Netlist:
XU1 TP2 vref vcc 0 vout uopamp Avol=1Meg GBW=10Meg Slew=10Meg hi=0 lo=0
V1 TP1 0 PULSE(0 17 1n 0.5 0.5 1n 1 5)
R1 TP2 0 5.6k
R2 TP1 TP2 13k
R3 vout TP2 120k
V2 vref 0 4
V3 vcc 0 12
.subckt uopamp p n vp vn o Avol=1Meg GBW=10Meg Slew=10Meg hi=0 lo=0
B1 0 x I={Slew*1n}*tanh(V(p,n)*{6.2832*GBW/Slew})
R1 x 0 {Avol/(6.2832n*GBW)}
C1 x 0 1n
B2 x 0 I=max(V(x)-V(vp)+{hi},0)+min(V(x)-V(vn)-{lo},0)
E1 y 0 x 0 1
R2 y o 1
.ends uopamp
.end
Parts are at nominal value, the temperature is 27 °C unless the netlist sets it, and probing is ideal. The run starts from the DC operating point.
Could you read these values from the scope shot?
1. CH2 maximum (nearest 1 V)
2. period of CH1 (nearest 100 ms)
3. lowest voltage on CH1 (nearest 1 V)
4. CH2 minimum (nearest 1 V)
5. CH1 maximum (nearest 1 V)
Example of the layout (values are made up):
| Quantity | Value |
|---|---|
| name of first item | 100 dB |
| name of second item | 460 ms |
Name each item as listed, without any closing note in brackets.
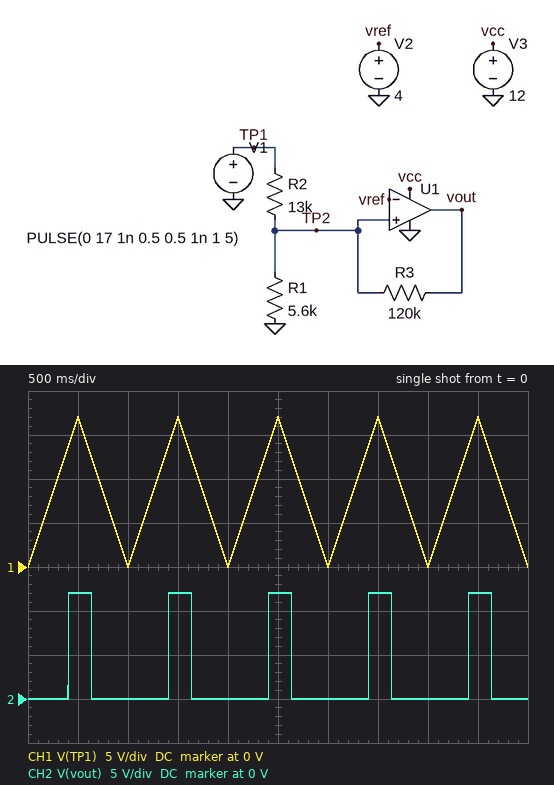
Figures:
| Quantity | Value |
|---|---|
| CH2 maximum | 12 V |
| period of CH1 | 1.0 s |
| lowest voltage on CH1 | 0 V |
| CH2 minimum | 0 V |
| CH1 maximum | 17 V |
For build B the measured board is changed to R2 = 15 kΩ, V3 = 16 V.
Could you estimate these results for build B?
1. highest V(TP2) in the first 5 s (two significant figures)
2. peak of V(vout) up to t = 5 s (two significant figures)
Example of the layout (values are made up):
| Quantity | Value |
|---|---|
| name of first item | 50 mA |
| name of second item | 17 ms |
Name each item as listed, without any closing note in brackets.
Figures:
| Quantity | Value |
|---|---|
| highest V(TP2) in the first 5 s | 5.0 V |
| peak of V(vout) up to t = 5 s | 16 V |
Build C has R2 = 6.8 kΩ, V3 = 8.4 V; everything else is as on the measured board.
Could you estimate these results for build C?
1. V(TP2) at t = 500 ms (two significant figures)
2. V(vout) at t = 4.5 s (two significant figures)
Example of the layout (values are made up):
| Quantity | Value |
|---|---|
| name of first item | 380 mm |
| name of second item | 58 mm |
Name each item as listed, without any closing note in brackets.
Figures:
| Quantity | Value |
|---|---|
| V(TP2) at t = 500 ms | 7.7 V |
| V(vout) at t = 4.5 s | 8.4 V |
